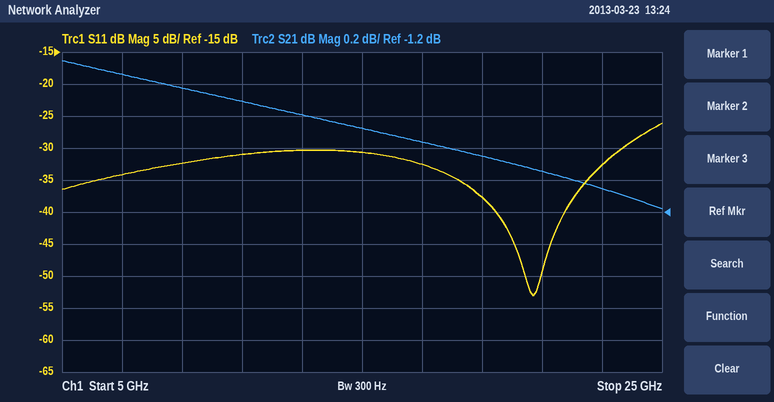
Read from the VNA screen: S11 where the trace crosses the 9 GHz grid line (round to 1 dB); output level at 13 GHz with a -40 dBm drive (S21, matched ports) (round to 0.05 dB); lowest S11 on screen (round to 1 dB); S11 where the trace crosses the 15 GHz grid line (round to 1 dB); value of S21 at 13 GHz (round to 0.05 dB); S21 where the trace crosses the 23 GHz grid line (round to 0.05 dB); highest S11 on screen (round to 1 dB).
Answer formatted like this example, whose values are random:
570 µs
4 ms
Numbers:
-32 dB
-40.60 dBm
-53 dB
-31 dB
-0.60 dB
-1.05 dB
-26 dB
